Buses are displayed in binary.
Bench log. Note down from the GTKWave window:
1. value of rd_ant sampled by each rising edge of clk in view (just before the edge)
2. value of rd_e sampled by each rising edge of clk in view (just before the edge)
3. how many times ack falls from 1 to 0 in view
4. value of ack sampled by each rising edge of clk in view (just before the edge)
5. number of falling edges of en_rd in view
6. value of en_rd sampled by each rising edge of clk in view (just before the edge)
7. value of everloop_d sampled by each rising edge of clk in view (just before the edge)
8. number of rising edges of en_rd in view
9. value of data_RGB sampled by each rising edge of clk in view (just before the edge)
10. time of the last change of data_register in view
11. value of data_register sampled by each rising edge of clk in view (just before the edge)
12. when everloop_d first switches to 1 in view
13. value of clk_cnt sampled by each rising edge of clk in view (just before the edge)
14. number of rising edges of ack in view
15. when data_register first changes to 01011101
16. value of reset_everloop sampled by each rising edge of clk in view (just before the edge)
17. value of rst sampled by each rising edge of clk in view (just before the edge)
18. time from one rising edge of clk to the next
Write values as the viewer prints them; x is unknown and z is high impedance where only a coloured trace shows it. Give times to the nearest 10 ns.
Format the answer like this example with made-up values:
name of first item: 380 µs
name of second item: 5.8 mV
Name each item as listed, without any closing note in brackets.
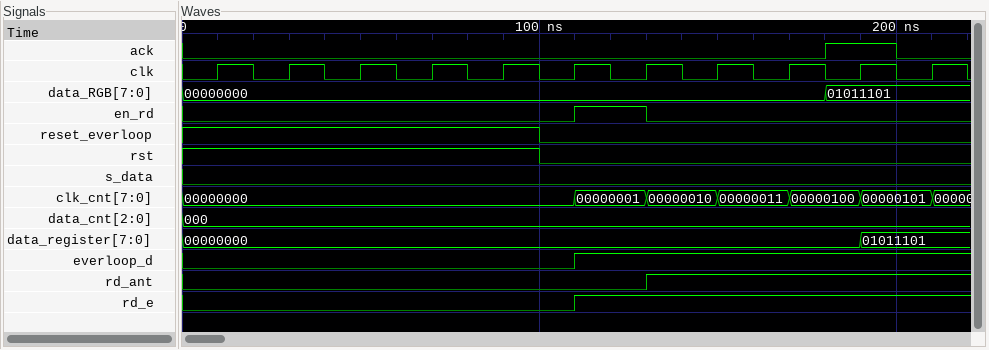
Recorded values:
value of rd_ant sampled by each rising edge of clk in view: 0 0 0 0 0 0 0 1 1 1 1
value of rd_e sampled by each rising edge of clk in view: 0 0 0 0 0 0 1 1 1 1 1
how many times ack falls from 1 to 0 in view: 1
value of ack sampled by each rising edge of clk in view: 0 0 0 0 0 0 0 0 0 1 0
number of falling edges of en_rd in view: 1
value of en_rd sampled by each rising edge of clk in view: 0 0 0 0 0 0 1 0 0 0 0
value of everloop_d sampled by each rising edge of clk in view: 0 0 0 0 0 0 1 1 1 1 1
number of rising edges of en_rd in view: 1
value of data_RGB sampled by each rising edge of clk in view: 00000000, 00000000, 00000000, 00000000, 00000000, 00000000, 00000000, 00000000, 00000000, 01011101, 01011101
time of the last change of data_register in view: 190 ns
value of data_register sampled by each rising edge of clk in view: 00000000, 00000000, 00000000, 00000000, 00000000, 00000000, 00000000, 00000000, 00000000, 00000000, 01011101
when everloop_d first switches to 1 in view: 110 ns
value of clk_cnt sampled by each rising edge of clk in view: 00000000, 00000000, 00000000, 00000000, 00000000, 00000000, 00000001, 00000010, 00000011, 00000100, 00000101
number of rising edges of ack in view: 1
when data_register first changes to 01011101: 190 ns
value of reset_everloop sampled by each rising edge of clk in view: 1 1 1 1 1 0 0 0 0 0 0
value of rst sampled by each rising edge of clk in view: 1 1 1 1 1 0 0 0 0 0 0
time from one rising edge of clk to the next: 20 ns
